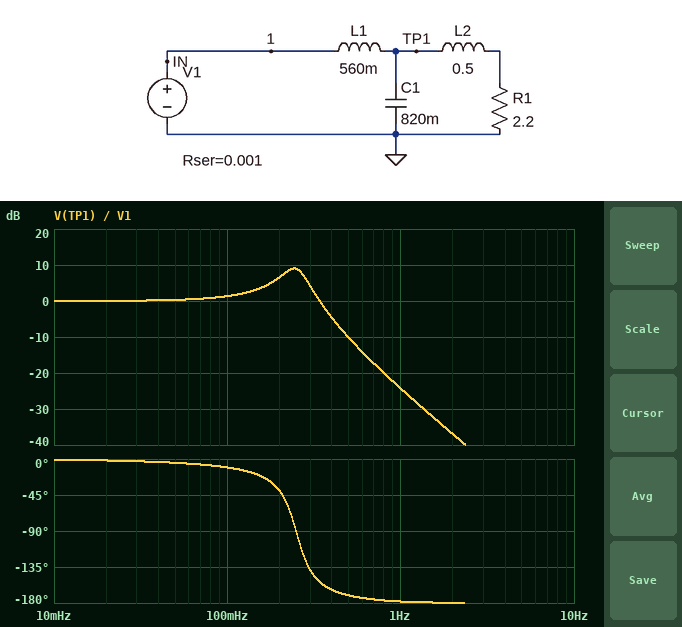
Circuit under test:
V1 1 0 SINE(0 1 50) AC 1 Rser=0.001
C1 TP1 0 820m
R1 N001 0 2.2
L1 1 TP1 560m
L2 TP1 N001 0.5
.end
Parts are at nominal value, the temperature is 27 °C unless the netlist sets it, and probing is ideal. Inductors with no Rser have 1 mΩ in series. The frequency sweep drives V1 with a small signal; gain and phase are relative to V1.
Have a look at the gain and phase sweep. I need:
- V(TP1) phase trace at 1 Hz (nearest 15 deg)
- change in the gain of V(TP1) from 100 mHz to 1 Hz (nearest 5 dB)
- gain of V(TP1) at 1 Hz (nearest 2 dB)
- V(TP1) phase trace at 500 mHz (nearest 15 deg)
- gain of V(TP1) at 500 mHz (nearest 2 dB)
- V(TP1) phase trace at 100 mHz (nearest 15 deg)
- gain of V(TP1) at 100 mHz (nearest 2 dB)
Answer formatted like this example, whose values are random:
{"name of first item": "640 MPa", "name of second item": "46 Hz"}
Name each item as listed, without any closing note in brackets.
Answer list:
{"V(TP1) phase trace at 1 Hz": "-180 deg", "change in the gain of V(TP1) from 100 mHz to 1 Hz": "-25 dB", "gain of V(TP1) at 1 Hz": "-24 dB", "V(TP1) phase trace at 500 mHz": "-165 deg", "gain of V(TP1) at 500 mHz": "-10 dB", "V(TP1) phase trace at 100 mHz": "-15 deg", "gain of V(TP1) at 100 mHz": "2 dB"}
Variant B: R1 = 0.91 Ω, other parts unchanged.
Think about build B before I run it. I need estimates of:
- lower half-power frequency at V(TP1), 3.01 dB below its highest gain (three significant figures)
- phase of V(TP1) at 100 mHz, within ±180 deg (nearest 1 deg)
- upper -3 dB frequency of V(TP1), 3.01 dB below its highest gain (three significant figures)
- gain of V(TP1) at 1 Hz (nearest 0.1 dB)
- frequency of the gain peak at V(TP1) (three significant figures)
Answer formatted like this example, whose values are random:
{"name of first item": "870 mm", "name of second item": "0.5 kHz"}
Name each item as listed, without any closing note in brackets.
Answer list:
{"lower half-power frequency at V(TP1), 3.01 dB below its highest gain": "210 mHz", "phase of V(TP1) at 100 mHz, within ±180 deg": "-20 deg", "upper -3 dB frequency of V(TP1), 3.01 dB below its highest gain": "351 mHz", "gain of V(TP1) at 1 Hz": "-24.1 dB", "frequency of the gain peak at V(TP1)": "294 mHz"}
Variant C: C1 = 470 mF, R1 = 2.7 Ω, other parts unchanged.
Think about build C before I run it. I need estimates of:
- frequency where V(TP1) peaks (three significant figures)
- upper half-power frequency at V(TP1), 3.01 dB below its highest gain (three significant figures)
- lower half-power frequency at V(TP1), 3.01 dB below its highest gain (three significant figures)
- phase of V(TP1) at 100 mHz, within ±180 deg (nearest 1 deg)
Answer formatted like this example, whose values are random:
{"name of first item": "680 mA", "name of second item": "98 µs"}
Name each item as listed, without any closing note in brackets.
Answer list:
{"frequency where V(TP1) peaks": "323 mHz", "upper half-power frequency at V(TP1), 3.01 dB below its highest gain": "381 mHz", "lower half-power frequency at V(TP1), 3.01 dB below its highest gain": "251 mHz", "phase of V(TP1) at 100 mHz, within ±180 deg": "-8 deg"}
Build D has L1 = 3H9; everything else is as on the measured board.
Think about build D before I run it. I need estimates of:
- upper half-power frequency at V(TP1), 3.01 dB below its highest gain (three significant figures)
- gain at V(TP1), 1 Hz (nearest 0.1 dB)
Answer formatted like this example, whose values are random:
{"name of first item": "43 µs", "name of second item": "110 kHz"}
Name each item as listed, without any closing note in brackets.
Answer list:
{"upper half-power frequency at V(TP1), 3.01 dB below its highest gain": "111 mHz", "gain at V(TP1), 1 Hz": "-41.6 dB"}
